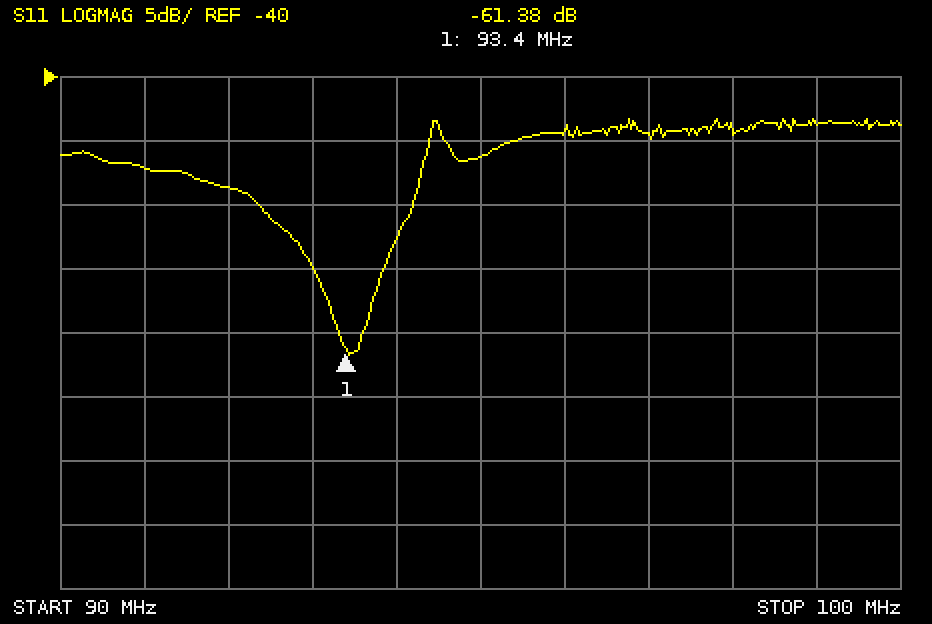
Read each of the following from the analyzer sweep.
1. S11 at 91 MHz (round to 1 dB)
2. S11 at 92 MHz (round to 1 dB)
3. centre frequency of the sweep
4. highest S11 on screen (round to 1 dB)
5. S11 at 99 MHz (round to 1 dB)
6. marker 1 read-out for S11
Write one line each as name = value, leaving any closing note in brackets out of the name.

S11 at 91 MHz = -47 dB
S11 at 92 MHz = -49 dB
centre frequency of the sweep = 95 MHz
highest S11 on screen = -43 dB
S11 at 99 MHz = -44 dB
marker 1 read-out for S11 = -61.38 dB
